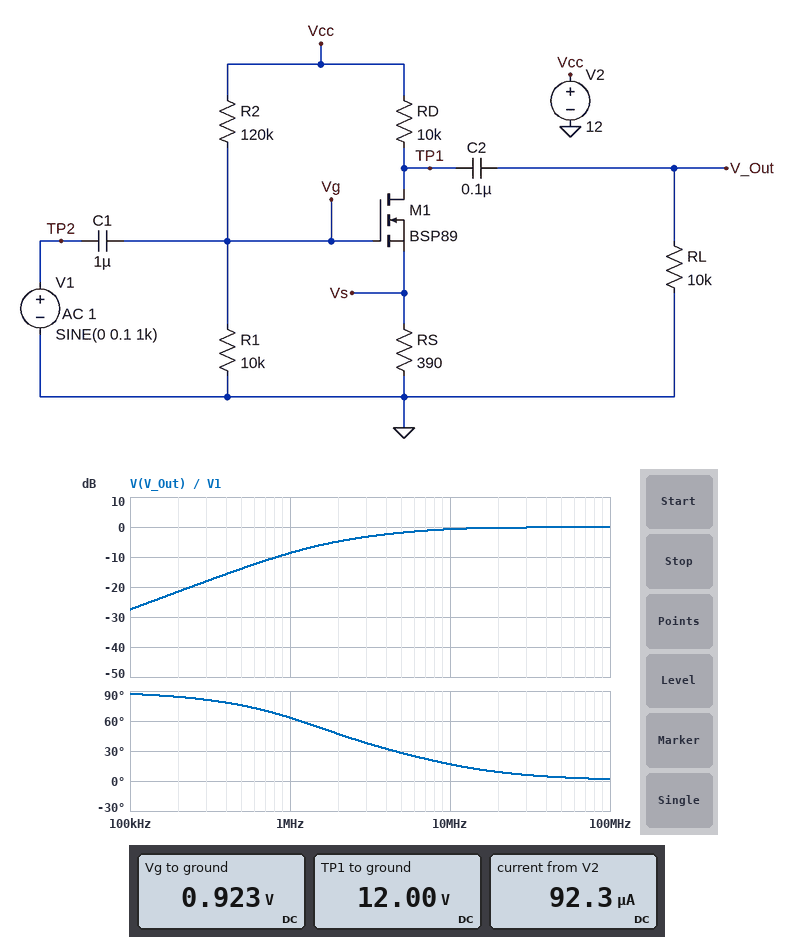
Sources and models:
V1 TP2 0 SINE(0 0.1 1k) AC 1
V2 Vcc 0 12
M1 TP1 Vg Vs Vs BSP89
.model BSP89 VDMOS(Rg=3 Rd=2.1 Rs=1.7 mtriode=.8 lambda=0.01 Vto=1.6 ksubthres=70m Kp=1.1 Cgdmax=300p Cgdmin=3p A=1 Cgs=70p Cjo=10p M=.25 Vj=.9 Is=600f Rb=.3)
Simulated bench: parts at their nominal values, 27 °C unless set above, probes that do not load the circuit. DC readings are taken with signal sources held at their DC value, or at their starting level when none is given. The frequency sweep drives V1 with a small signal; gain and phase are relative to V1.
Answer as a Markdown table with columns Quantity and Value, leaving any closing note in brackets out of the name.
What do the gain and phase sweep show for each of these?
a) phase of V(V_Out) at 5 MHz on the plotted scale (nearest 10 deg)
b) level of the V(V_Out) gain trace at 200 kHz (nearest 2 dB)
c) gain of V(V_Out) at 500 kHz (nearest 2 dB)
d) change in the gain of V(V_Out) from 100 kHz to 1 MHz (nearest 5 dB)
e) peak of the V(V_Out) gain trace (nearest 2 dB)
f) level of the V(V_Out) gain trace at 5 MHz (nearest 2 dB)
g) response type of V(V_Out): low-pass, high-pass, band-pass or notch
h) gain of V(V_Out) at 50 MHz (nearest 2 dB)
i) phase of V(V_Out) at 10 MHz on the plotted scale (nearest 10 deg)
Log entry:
| Quantity | Value |
|---|---|
| phase of V(V_Out) at 5 MHz on the plotted scale | 30 deg |
| level of the V(V_Out) gain trace at 200 kHz | -22 dB |
| gain of V(V_Out) at 500 kHz | -14 dB |
| change in the gain of V(V_Out) from 100 kHz to 1 MHz | 20 dB |
| peak of the V(V_Out) gain trace | 0 dB |
| level of the V(V_Out) gain trace at 5 MHz | -2 dB |
| response type of V(V_Out): low-pass, high-pass, band-pass or notch | high-pass |
| gain of V(V_Out) at 50 MHz | 0 dB |
| phase of V(V_Out) at 10 MHz on the plotted scale | 20 deg |
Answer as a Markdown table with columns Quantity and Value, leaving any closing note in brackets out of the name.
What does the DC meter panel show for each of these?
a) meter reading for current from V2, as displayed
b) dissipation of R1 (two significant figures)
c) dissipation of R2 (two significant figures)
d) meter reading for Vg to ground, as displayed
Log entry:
| Quantity | Value |
|---|---|
| meter reading for current from V2, as displayed | 92.3 µA |
| dissipation of R1 | 85 µW |
| dissipation of R2 | 1.0 mW |
| meter reading for Vg to ground, as displayed | 0.923 V |
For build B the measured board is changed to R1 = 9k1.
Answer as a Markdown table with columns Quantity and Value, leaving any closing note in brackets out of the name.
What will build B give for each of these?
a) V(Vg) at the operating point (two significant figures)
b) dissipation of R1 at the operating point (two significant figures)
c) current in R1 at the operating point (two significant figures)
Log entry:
| Quantity | Value |
|---|---|
| V(Vg) at the operating point | 850 mV |
| dissipation of R1 at the operating point | 79 µW |
| current in R1 at the operating point | 93 µA |
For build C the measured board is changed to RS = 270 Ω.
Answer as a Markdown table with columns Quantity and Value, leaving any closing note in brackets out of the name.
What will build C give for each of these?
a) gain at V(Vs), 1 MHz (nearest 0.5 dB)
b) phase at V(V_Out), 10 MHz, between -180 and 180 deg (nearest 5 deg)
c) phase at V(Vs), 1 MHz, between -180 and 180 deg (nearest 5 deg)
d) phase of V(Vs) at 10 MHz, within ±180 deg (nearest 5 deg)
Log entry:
| Quantity | Value |
|---|---|
| gain at V(Vs), 1 MHz | -18.5 dB |
| phase at V(V_Out), 10 MHz, between -180 and 180 deg | 20 deg |
| phase at V(Vs), 1 MHz, between -180 and 180 deg | 85 deg |
| phase of V(Vs) at 10 MHz, within ±180 deg | 40 deg |
